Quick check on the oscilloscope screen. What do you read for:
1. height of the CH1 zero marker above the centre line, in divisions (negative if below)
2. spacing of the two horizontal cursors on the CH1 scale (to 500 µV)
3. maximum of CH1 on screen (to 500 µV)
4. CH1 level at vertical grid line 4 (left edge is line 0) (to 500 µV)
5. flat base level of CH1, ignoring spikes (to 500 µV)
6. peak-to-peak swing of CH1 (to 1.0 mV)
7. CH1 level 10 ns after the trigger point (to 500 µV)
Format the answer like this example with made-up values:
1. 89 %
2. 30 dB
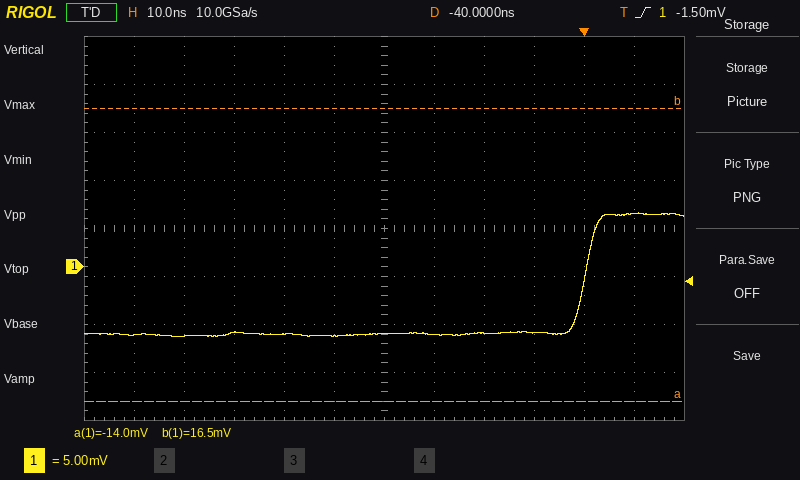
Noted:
1. -0.8 div
2. 30.5 mV
3. 5.5 mV
4. -7.0 mV
5. -7.0 mV
6. 13.0 mV
7. 5.5 mV
